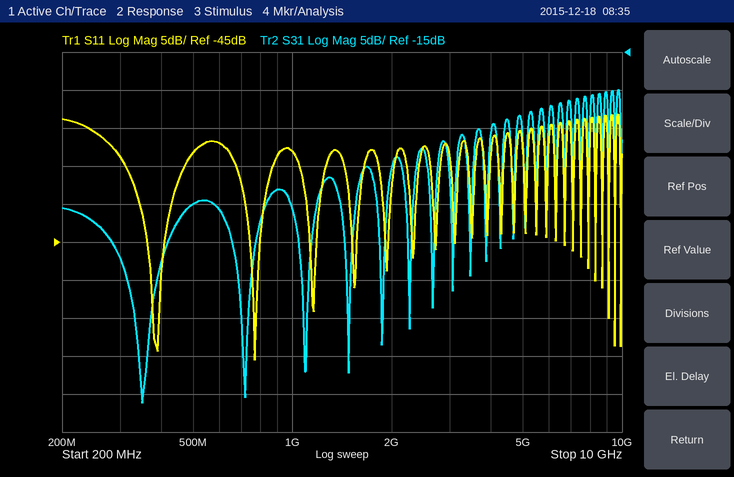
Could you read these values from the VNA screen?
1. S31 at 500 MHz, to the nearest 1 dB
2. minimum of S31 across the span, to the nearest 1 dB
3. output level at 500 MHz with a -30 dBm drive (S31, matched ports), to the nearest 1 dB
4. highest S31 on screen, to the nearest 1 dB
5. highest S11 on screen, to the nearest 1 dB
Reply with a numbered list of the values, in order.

1. -35 dB
2. -61 dB
3. -65 dBm
4. -20 dB
5. -28 dB
